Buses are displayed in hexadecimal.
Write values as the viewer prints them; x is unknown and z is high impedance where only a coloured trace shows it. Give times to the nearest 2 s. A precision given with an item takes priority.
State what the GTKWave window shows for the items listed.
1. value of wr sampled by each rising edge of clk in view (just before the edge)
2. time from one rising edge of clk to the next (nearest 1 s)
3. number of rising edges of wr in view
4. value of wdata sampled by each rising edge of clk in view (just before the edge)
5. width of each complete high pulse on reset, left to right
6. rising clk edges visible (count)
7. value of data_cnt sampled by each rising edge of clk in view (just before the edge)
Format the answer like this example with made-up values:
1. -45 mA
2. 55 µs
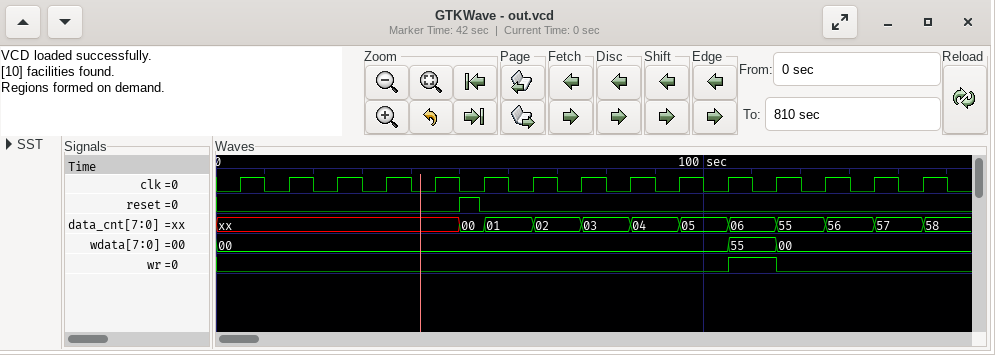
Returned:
1. 0 0 0 0 0 0 0 0 0 0 0 1 0 0 0
2. 10 s
3. 1
4. 00, 00, 00, 00, 00, 00, 00, 00, 00, 00, 00, 55, 00, 00, 00
5. 4 s
6. 15
7. xx, xx, xx, xx, xx, 00, 01, 02, 03, 04, 05, 06, 55, 56, 57
